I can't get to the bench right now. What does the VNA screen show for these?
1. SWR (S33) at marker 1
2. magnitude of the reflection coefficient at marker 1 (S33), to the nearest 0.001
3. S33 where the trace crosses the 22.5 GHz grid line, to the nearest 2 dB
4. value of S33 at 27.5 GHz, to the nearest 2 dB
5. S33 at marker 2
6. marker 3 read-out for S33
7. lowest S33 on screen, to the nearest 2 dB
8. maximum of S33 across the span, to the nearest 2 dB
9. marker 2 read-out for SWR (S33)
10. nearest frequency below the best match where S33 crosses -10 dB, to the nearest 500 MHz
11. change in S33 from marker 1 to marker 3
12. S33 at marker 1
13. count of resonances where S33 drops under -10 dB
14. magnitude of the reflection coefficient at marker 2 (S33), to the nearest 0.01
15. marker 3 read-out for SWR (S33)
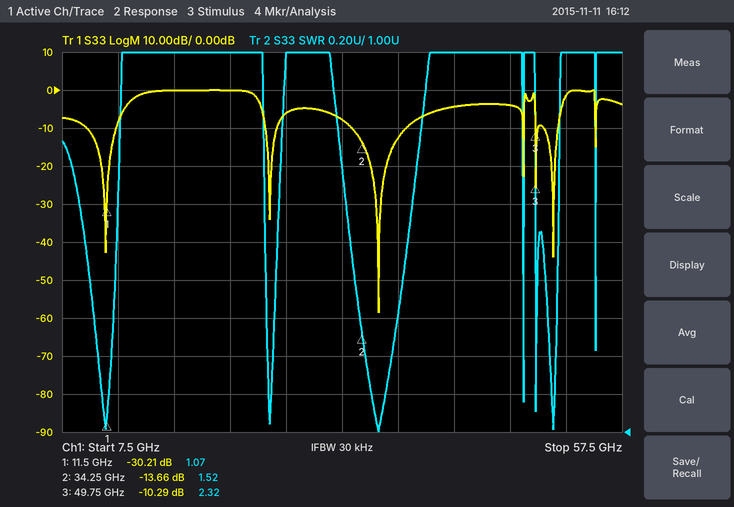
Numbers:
1.07
0.031
0 dB
-6 dB
-13.66 dB
-10.29 dB
-58 dB
0 dB
1.52
33.5 GHz
19.92 dB
-30.21 dB
7
0.21
2.32
